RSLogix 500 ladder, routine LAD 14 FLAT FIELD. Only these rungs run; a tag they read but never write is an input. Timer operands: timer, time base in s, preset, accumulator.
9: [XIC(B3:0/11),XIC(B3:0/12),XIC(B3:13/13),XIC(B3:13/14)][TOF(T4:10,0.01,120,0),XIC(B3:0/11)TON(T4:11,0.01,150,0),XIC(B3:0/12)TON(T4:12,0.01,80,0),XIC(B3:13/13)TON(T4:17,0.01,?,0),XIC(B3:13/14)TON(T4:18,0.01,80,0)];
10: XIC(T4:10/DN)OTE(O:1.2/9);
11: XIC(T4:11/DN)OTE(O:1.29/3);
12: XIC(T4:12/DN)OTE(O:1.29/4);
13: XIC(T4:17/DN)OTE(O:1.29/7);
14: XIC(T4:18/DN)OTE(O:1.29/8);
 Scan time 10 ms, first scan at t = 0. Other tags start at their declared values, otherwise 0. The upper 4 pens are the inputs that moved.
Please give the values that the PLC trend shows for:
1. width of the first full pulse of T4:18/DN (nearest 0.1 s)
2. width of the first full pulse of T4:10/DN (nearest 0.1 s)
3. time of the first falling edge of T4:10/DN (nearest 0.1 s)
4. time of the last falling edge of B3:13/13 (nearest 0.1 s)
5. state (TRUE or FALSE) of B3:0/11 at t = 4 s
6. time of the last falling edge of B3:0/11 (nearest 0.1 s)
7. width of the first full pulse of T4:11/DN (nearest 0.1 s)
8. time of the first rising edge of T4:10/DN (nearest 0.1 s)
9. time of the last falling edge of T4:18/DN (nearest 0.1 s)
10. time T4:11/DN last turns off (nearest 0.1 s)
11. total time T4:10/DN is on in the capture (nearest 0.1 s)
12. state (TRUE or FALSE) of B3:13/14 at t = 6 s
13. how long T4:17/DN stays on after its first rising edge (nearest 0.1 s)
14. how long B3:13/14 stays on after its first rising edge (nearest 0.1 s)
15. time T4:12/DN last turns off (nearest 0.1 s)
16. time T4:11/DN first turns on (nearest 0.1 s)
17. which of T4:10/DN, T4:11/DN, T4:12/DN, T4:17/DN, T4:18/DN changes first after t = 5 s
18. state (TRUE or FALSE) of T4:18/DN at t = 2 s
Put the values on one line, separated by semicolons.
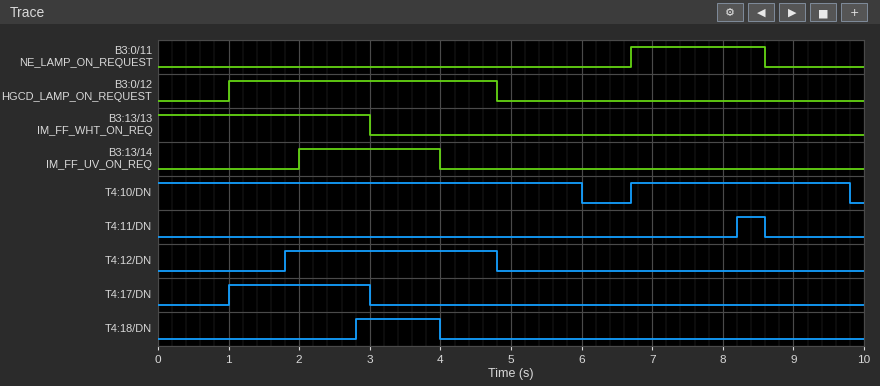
1.2 s; 3.1 s; 6.0 s; 3.0 s; FALSE; 8.6 s; 0.4 s; 6.7 s; 4.0 s; 8.6 s; 9.1 s; FALSE; 2.0 s; 2.0 s; 4.8 s; 8.2 s; T4:10/DN; FALSE
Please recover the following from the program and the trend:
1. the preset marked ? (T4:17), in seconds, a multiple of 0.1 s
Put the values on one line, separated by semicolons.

1.0 s
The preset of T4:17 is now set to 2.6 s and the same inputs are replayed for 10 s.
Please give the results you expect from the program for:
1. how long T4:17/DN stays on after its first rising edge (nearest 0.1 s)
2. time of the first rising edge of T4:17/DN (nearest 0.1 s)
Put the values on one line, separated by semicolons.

0.4 s; 2.6 s
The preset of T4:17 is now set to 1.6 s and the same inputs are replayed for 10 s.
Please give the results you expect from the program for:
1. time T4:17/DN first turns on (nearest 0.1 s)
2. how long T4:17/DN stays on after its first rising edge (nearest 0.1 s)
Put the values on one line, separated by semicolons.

1.6 s; 1.4 s
